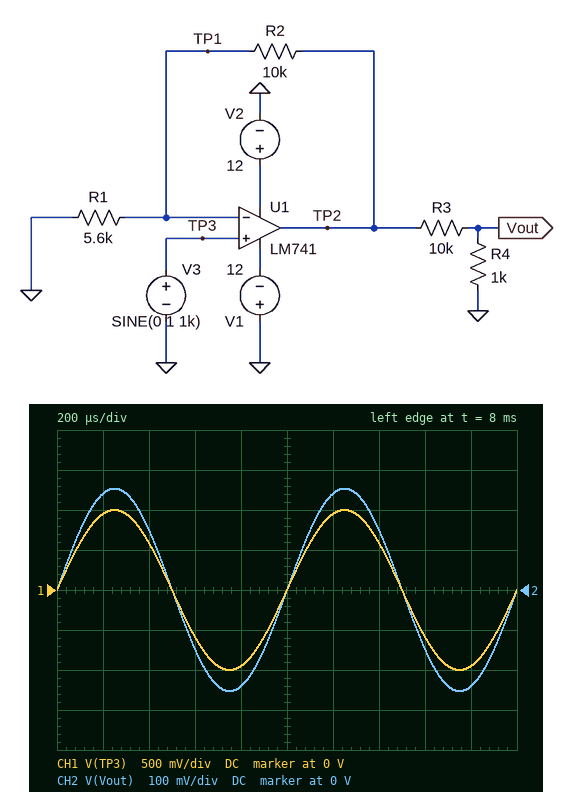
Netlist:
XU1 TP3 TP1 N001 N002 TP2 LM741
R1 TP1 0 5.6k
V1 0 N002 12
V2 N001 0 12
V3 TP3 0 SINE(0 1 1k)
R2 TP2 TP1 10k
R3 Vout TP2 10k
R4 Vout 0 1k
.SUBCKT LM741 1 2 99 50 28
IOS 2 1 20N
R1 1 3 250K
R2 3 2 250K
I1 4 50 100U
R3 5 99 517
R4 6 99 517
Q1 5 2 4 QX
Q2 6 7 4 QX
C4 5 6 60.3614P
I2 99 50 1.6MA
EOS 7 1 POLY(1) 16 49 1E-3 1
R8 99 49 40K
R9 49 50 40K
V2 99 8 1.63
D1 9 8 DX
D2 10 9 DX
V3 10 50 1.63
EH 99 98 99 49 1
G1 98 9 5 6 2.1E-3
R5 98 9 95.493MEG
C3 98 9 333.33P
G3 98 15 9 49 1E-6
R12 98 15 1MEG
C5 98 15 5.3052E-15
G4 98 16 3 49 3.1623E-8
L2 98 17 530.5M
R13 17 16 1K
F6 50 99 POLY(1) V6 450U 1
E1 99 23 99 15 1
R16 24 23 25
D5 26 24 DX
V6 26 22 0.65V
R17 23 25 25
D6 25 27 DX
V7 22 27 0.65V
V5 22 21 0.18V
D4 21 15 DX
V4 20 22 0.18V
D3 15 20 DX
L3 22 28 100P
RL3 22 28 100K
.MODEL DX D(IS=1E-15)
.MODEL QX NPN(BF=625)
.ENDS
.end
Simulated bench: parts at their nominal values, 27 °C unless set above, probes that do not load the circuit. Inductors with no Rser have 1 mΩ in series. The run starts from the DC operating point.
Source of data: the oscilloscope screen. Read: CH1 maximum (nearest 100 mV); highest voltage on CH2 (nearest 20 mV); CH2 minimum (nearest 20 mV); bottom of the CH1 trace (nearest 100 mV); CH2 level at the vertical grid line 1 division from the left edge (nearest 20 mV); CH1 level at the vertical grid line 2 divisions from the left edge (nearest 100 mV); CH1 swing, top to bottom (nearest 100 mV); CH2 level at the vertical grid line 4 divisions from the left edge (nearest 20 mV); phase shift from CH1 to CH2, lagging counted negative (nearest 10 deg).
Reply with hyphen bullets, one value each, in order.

- 1.0 V
- 260 mV
- -260 mV
- -1.0 V
- 240 mV
- 600 mV
- 2.0 V
- -240 mV
- 0 deg
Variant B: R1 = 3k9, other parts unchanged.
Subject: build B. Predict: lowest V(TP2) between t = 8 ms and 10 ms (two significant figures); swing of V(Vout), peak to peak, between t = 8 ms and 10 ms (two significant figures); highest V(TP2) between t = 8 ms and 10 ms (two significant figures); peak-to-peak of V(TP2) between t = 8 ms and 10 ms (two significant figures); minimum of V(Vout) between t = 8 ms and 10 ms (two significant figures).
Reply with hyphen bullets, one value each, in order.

- -3.6 V
- 650 mV
- 3.6 V
- 7.1 V
- -320 mV
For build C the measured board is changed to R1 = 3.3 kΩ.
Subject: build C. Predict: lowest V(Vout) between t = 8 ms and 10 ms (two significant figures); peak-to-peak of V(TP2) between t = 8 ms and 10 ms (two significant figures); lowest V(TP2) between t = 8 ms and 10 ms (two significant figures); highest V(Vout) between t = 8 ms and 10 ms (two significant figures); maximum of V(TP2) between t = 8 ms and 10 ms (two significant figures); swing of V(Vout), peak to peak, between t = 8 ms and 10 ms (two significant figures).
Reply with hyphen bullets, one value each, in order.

- -370 mV
- 8.1 V
- -4.0 V
- 370 mV
- 4.0 V
- 730 mV
